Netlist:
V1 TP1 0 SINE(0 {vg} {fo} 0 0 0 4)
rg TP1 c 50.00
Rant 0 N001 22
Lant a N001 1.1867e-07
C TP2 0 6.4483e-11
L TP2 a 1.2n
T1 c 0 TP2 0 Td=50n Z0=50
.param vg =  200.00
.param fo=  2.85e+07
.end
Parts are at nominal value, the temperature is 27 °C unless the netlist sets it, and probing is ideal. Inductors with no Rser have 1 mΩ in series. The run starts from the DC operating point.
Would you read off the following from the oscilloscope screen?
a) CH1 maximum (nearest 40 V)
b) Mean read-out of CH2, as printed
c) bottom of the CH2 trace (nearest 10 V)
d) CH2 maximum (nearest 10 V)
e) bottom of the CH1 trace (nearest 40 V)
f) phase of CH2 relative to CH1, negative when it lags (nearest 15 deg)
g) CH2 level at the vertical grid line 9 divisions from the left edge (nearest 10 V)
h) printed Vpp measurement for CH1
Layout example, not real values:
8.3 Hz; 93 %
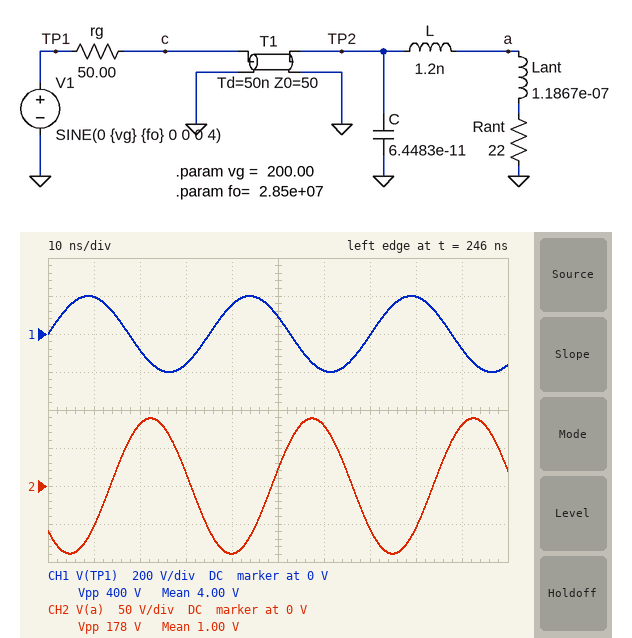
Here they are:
200 V; 1.00 V; -90 V; 90 V; -200 V; -135 deg; 80 V; 400 V
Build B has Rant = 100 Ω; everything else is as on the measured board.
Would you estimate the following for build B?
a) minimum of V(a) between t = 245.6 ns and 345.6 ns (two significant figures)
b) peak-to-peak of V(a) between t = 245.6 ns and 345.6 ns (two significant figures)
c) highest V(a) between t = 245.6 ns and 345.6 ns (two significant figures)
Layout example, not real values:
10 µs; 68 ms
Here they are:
-130 V; 260 V; 130 V
